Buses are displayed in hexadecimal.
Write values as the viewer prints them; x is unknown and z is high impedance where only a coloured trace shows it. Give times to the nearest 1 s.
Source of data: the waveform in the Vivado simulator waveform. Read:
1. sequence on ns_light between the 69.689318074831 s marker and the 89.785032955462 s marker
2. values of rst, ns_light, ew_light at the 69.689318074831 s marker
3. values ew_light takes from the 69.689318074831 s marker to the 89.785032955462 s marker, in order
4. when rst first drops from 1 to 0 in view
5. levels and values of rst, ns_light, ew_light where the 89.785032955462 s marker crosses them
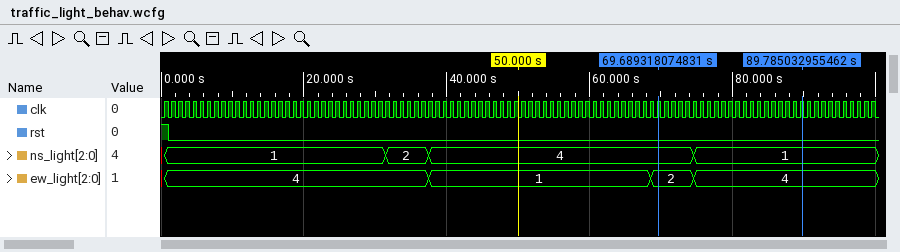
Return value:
4, 1
rst=0, ns_light=4, ew_light=2
2, 4
1 s
rst=0, ns_light=1, ew_light=4
